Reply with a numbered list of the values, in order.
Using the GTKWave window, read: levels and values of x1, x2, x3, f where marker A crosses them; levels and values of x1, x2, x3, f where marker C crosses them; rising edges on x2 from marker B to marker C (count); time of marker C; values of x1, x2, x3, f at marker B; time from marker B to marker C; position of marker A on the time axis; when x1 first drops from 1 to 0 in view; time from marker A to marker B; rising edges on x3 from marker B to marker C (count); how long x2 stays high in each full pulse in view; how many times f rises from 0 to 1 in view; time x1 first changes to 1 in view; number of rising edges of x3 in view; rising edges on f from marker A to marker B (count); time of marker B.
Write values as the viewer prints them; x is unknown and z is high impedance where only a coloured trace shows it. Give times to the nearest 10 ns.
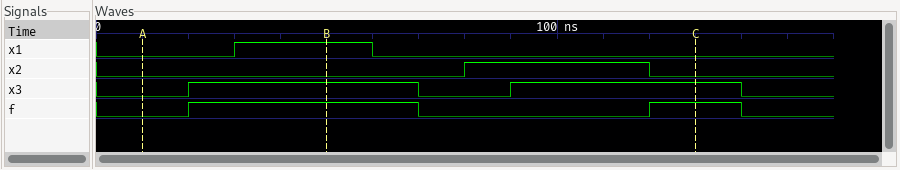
1. x1=0, x2=0, x3=0, f=0
2. x1=0, x2=0, x3=1, f=1
3. 1
4. 130 ns
5. x1=1, x2=0, x3=1, f=1
6. 80 ns
7. 10 ns
8. 60 ns
9. 40 ns
10. 1
11. 40 ns
12. 2
13. 30 ns
14. 2
15. 1
16. 50 ns
